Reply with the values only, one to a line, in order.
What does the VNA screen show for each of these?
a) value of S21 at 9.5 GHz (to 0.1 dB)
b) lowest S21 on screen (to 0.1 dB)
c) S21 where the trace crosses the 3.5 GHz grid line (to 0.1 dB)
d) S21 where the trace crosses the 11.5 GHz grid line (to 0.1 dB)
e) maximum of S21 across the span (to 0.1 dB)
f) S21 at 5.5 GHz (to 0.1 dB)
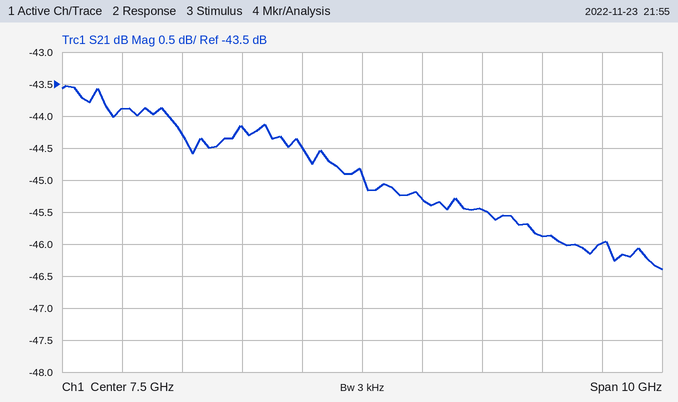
-45.5 dB
-46.4 dB
-43.9 dB
-46.0 dB
-43.5 dB
-44.2 dB
